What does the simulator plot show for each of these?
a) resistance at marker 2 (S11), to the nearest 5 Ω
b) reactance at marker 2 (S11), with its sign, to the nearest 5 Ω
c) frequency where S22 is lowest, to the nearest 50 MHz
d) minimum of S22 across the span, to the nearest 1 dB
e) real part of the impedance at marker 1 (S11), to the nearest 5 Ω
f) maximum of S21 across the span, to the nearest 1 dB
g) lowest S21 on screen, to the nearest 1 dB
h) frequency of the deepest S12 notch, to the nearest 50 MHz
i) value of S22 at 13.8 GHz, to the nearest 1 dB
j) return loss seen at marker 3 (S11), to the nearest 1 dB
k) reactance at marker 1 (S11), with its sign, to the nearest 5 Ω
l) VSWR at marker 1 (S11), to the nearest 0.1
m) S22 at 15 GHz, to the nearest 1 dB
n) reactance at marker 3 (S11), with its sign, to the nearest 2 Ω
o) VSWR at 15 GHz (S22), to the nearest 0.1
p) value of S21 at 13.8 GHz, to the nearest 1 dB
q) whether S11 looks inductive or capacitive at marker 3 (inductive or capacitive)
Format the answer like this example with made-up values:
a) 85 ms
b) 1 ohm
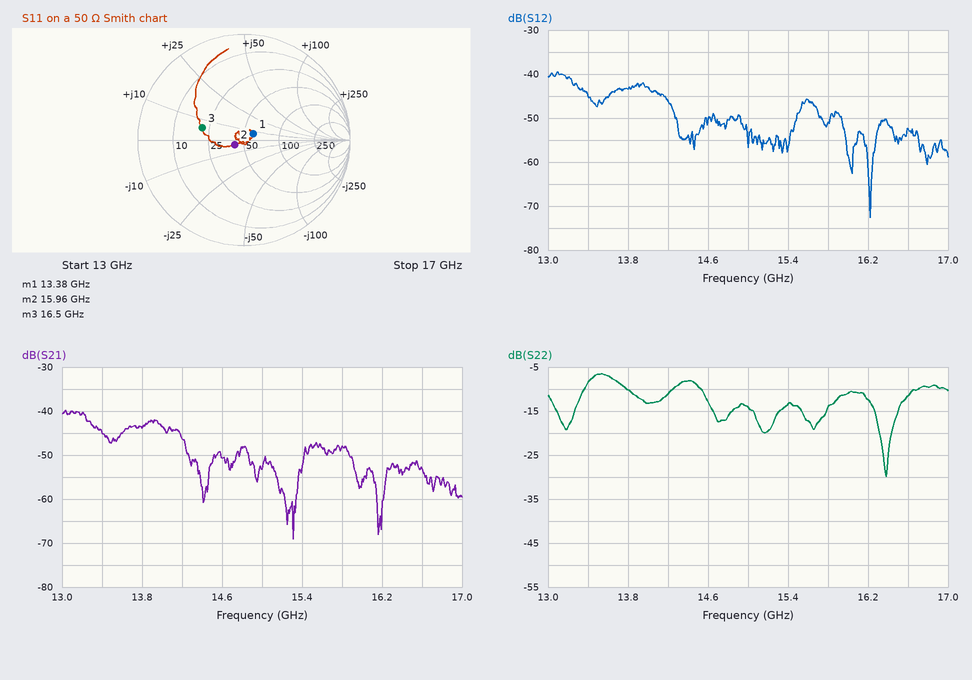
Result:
a) 40 Ω
b) -5 Ω
c) 16.40 GHz
d) -30 dB
e) 60 Ω
f) -40 dB
g) -69 dB
h) 16.20 GHz
i) -10 dB
j) 8 dB
k) +5 Ω
l) 1.2
m) -14 dB
n) +6 Ω
o) 1.5
p) -44 dB
q) inductive
